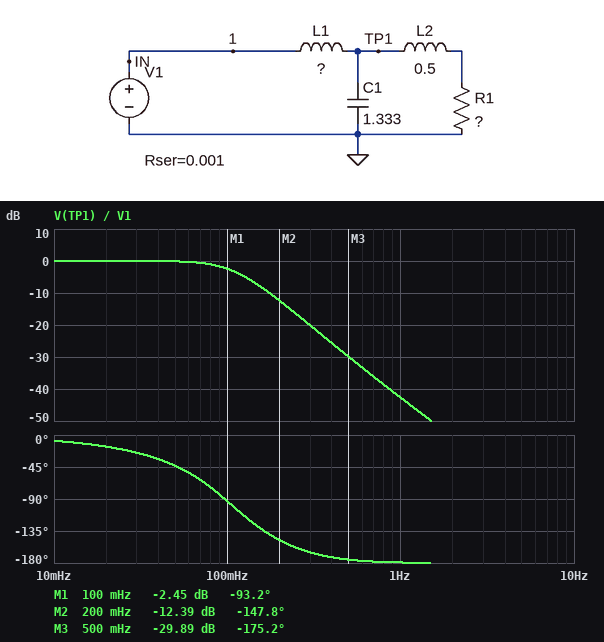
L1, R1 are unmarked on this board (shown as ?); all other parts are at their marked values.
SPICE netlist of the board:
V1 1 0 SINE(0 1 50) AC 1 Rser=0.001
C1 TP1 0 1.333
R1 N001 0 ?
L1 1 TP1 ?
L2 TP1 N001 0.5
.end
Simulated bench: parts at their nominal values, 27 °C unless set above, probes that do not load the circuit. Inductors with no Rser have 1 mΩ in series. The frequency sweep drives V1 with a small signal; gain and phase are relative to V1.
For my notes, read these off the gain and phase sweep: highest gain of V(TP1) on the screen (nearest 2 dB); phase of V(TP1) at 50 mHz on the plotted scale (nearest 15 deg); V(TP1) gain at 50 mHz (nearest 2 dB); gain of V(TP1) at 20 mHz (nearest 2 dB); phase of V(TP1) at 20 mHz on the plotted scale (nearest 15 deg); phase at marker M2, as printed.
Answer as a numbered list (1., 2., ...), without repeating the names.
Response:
1. 0 dB
2. -45 deg
3. 0 dB
4. 0 dB
5. -15 deg
6. -147.8 deg
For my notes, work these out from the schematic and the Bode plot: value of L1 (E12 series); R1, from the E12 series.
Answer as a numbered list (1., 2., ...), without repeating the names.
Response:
1. 2.7 H
2. 1.2 Ω
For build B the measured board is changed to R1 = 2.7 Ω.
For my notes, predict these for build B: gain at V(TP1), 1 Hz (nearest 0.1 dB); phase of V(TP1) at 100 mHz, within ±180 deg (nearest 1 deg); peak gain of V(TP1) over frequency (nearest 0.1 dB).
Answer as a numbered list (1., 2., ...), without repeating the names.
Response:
1. -42.8 dB
2. -119 deg
3. 5.7 dB
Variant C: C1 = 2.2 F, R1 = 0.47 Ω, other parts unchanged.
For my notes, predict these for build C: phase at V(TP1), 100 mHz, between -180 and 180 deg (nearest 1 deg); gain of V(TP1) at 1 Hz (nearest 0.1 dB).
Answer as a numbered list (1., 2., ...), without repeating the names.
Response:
1. -83 deg
2. -47.2 dB
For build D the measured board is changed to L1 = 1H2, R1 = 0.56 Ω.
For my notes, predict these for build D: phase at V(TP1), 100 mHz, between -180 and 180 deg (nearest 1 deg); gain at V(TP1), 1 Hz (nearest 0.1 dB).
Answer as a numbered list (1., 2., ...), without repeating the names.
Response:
1. -47 deg
2. -35.5 dB
